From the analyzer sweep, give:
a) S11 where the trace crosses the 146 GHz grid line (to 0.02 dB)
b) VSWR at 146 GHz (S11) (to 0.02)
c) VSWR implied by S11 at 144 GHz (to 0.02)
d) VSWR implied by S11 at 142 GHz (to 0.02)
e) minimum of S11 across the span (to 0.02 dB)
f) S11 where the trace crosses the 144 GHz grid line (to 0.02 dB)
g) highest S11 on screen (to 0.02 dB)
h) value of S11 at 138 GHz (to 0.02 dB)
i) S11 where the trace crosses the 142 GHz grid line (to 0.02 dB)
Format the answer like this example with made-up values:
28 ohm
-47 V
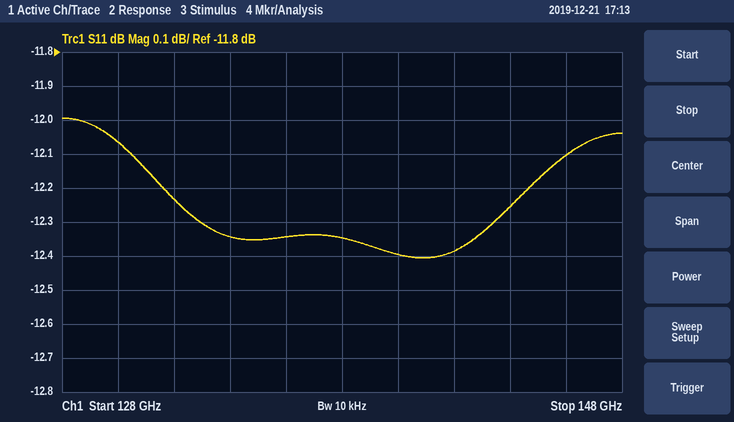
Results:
-12.10 dB
1.66
1.64
1.64
-12.40 dB
-12.26 dB
-12.00 dB
-12.34 dB
-12.38 dB
